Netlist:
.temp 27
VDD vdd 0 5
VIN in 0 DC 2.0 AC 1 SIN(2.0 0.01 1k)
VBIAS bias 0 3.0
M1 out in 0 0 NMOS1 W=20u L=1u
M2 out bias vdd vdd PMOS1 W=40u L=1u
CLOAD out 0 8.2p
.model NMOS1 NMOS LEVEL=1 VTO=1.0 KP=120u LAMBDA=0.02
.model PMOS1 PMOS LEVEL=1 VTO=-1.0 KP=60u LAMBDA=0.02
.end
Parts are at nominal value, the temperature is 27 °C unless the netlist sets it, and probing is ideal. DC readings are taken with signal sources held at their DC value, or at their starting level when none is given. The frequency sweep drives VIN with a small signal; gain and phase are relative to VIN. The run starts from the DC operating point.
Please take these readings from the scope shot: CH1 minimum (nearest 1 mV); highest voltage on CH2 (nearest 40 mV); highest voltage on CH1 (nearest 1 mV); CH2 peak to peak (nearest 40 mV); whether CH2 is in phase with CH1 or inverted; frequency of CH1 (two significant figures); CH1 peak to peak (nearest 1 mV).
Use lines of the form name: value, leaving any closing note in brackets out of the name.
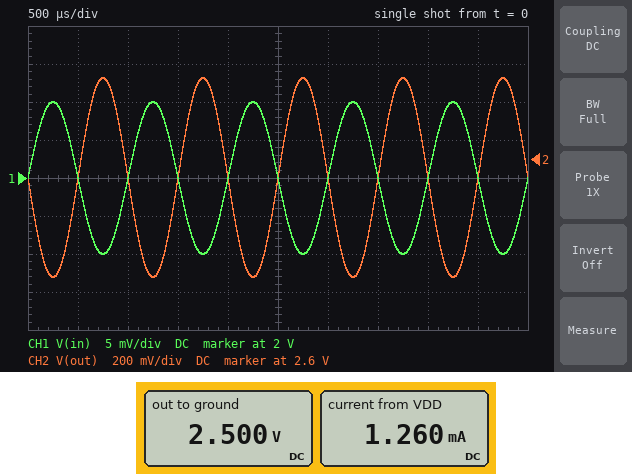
CH1 minimum: 1.990 V
highest voltage on CH2: 3.04 V
highest voltage on CH1: 2.010 V
CH2 peak to peak: 1.04 V
whether CH2 is in phase with CH1 or inverted: inverted
frequency of CH1: 1.0 kHz
CH1 peak to peak: 20 mV
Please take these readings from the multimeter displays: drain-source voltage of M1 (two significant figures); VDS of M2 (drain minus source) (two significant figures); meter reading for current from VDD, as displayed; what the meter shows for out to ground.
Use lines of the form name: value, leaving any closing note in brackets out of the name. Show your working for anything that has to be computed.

drain-source voltage of M1: 2.5 V = 2.5 V
VDS of M2 (drain minus source): 2.5 V - 5 V = -2.5 V
meter reading for current from VDD, as displayed: 1.260 mA
what the meter shows for out to ground: 2.500 V
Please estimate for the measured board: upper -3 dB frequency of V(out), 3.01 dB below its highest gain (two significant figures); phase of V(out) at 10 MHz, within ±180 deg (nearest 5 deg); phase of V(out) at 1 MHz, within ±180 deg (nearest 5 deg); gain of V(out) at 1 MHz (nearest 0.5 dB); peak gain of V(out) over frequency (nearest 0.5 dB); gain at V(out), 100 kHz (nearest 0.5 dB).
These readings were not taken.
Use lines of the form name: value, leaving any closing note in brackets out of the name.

upper -3 dB frequency of V(out), 3.01 dB below its highest gain: 930 kHz
phase of V(out) at 10 MHz, within ±180 deg: 95 deg
phase of V(out) at 1 MHz, within ±180 deg: 135 deg
gain of V(out) at 1 MHz: 31.0 dB
peak gain of V(out) over frequency: 34.5 dB
gain at V(out), 100 kHz: 34.5 dB
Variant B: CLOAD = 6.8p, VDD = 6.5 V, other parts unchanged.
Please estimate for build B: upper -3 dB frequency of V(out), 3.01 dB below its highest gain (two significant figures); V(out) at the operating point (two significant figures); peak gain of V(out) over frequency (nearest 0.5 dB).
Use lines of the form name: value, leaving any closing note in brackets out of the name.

upper -3 dB frequency of V(out), 3.01 dB below its highest gain: 130 MHz
V(out) at the operating point: 6.3 V
peak gain of V(out) over frequency: -6.0 dB
